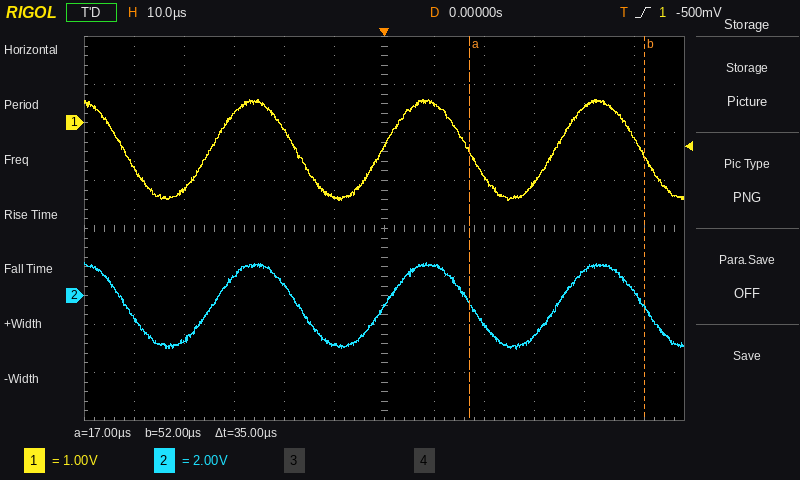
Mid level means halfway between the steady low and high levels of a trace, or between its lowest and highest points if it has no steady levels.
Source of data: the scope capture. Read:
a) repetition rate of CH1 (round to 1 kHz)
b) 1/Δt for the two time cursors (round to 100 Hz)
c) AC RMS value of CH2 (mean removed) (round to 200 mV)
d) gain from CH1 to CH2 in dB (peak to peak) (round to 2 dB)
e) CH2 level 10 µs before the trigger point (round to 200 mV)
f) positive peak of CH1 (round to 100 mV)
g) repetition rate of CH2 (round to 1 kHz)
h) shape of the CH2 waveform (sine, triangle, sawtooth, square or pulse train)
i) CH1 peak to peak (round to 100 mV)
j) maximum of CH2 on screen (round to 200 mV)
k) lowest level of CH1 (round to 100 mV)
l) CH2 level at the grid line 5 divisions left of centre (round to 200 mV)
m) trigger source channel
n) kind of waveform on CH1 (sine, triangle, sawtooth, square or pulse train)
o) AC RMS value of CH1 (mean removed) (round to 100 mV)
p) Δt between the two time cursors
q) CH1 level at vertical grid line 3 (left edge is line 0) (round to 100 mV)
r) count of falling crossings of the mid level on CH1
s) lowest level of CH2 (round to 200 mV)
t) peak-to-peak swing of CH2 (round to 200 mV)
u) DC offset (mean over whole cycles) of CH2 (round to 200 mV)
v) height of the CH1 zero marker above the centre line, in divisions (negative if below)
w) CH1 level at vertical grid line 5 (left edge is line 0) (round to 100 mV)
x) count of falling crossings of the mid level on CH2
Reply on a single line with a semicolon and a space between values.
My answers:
29 kHz; 28.6 kHz; 1.2 V; 4 dB; -2.0 V; 500 mV; 29 kHz; sine; 2.1 V; 1.4 V; -1.6 V; -1.0 V; CH1; sine; 700 mV; 35 µs; 200 mV; 4; -2.2 V; 3.6 V; -400 mV; +2.2 div; -1.5 V; 4
